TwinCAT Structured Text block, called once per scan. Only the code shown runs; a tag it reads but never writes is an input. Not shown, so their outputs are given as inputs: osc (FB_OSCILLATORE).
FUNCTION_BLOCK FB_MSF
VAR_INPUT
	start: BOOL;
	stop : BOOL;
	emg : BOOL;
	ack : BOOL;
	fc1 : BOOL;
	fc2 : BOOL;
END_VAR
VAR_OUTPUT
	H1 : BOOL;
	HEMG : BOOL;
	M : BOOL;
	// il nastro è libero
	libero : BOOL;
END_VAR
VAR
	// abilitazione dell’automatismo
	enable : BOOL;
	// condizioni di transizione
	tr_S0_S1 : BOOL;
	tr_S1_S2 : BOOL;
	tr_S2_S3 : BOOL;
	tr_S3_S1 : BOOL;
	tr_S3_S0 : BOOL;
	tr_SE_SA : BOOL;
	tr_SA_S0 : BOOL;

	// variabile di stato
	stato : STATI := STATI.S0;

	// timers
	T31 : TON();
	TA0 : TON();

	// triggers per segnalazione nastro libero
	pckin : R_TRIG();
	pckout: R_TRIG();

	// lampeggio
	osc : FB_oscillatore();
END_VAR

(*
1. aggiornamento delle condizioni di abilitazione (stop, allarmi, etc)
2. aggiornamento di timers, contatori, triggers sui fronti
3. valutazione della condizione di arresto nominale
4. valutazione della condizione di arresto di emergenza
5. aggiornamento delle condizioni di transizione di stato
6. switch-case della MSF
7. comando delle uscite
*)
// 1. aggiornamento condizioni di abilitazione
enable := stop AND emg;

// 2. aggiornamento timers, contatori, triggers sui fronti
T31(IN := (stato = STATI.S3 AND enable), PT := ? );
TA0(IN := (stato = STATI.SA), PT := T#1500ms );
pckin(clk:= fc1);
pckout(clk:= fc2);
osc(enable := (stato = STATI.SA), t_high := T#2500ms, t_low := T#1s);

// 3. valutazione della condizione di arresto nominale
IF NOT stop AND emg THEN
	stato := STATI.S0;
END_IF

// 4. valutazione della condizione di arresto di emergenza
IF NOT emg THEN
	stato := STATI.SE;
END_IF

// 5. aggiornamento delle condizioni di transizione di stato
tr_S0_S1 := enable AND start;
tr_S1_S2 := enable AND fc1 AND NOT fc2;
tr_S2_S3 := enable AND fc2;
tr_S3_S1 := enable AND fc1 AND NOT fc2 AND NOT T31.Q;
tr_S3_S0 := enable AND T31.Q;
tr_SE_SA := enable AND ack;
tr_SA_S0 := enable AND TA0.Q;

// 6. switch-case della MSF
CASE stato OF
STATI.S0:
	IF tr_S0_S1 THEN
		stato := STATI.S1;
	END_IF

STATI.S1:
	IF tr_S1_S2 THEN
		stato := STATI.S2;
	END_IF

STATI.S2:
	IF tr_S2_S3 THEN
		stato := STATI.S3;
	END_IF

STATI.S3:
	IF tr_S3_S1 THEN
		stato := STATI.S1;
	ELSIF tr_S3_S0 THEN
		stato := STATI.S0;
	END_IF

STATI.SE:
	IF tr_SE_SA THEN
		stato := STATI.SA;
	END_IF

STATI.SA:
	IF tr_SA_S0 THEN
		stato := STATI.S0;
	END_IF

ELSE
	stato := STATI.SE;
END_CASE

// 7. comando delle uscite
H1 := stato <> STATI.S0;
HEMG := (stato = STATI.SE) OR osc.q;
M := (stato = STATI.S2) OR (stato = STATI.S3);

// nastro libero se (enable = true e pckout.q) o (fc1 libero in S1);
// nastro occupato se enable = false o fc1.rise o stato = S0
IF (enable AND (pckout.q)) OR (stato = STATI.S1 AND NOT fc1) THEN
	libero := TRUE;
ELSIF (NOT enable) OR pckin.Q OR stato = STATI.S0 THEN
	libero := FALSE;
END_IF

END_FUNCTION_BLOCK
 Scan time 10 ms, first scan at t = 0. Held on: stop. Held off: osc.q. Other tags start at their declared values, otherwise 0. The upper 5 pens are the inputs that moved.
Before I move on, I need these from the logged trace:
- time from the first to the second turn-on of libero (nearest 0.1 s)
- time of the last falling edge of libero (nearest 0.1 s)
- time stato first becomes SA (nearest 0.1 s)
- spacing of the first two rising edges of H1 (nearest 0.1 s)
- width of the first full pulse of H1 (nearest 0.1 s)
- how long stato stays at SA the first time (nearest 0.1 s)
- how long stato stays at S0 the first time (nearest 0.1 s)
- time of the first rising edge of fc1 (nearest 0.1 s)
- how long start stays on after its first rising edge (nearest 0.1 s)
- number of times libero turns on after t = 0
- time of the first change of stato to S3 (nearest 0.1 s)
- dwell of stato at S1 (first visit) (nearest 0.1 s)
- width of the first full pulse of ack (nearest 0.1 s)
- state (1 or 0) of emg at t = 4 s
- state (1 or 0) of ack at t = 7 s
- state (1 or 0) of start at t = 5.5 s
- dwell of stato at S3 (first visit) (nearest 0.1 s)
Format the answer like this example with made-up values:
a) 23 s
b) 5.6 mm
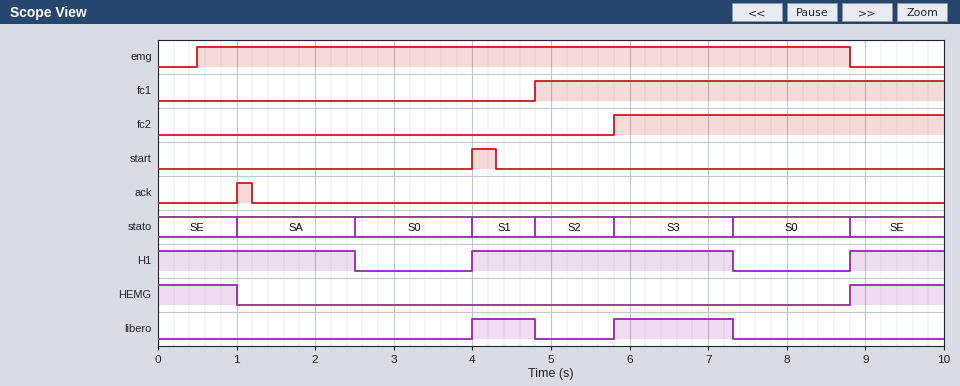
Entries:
a) 1.8 s
b) 7.3 s
c) 1.0 s
d) 4.8 s
e) 3.3 s
f) 1.5 s
g) 1.5 s
h) 4.8 s
i) 0.3 s
j) 2
k) 5.8 s
l) 0.8 s
m) 0.2 s
n) 1
o) 0
p) 0
q) 1.5 s
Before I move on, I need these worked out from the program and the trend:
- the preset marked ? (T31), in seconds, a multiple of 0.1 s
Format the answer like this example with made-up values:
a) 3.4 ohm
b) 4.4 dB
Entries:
a) 1.5 s
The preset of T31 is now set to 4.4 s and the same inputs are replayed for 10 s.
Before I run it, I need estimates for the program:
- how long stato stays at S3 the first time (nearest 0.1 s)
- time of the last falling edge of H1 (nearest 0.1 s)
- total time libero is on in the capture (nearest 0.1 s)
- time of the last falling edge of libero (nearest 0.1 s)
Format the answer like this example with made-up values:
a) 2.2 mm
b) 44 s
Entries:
a) 3.0 s
b) 2.5 s
c) 3.8 s
d) 8.8 s
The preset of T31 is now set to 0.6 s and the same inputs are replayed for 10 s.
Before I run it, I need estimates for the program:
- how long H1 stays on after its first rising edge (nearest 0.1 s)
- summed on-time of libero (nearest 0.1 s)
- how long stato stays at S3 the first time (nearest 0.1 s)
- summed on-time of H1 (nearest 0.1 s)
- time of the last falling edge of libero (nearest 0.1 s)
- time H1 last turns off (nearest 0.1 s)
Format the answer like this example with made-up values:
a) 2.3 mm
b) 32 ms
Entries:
a) 2.4 s
b) 1.4 s
c) 0.6 s
d) 6.1 s
e) 6.4 s
f) 6.4 s
